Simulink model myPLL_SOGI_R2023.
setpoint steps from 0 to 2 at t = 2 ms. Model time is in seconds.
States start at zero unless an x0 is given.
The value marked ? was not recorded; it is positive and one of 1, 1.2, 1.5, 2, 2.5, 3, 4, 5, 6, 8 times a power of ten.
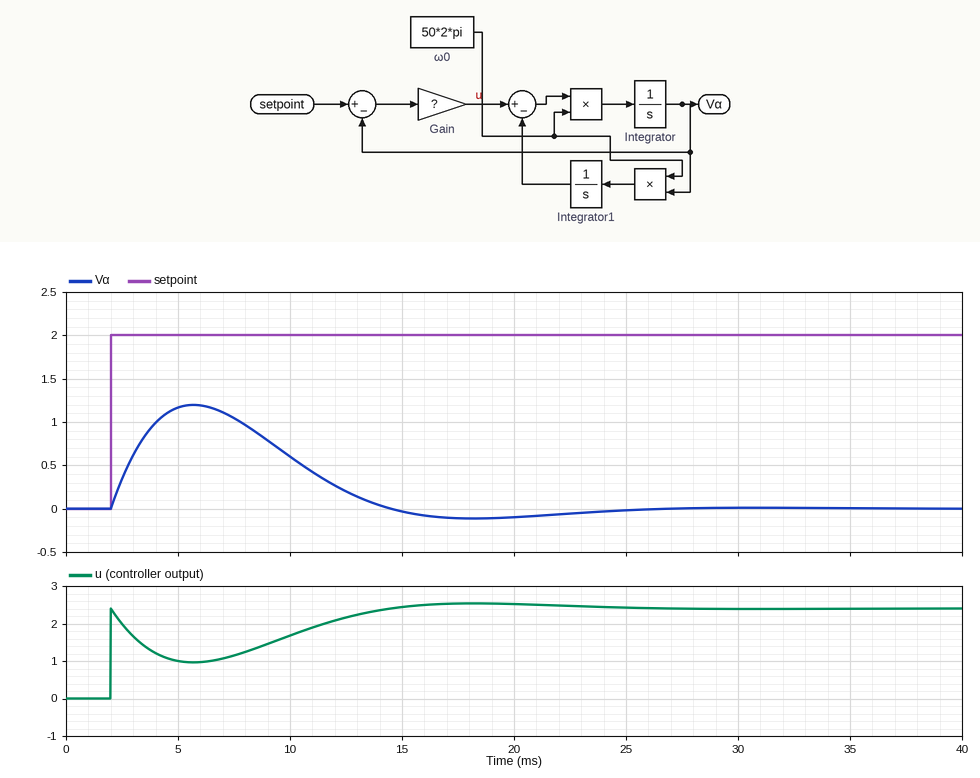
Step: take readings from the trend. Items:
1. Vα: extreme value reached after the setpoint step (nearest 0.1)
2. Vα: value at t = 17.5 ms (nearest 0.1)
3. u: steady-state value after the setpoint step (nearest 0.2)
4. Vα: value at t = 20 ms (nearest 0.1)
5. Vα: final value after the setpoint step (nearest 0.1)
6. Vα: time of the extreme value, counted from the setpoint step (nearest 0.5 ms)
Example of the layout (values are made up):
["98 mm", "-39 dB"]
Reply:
["1.2", "-0.1", "2.4", "-0.1", "0.0", "3.5 ms"]
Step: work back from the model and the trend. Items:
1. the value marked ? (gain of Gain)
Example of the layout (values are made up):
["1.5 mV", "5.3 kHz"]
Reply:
["1.2"]
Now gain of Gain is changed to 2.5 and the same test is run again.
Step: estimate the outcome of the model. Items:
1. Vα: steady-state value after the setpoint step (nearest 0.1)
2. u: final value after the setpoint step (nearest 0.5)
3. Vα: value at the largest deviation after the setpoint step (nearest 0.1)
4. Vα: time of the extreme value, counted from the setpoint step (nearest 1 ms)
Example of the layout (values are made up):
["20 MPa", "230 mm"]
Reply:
["0.0", "5.0", "1.6", "3 ms"]
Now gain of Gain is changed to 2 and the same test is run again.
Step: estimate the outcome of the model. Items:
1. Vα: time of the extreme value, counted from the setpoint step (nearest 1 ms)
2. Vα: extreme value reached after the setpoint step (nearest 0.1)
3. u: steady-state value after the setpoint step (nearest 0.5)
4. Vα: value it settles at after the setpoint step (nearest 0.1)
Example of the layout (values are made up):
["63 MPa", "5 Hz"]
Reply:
["3 ms", "1.5", "4.0", "0.0"]
